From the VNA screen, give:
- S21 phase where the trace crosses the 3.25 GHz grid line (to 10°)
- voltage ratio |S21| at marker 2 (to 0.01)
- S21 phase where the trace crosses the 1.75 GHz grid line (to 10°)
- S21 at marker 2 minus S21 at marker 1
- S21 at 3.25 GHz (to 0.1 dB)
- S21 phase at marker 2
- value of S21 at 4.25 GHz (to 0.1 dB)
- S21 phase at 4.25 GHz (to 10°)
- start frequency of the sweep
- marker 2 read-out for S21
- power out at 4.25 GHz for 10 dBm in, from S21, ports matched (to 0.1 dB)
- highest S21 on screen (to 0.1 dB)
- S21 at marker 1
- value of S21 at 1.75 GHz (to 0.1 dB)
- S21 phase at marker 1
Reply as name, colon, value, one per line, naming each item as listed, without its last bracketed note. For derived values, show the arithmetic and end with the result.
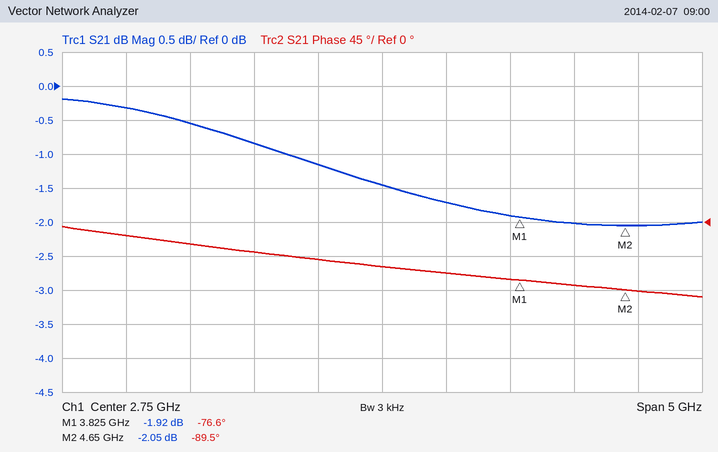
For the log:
S21 phase where the trace crosses the 3.25 GHz grid line: -70°
voltage ratio |S21| at marker 2: 10^(-2.05/20) ≈ 0.79
S21 phase where the trace crosses the 1.75 GHz grid line: -40°
S21 at marker 2 minus S21 at marker 1: -2.05 − (-1.92) = -0.13 dB
S21 at 3.25 GHz: -1.7 dB
S21 phase at marker 2: -89.5°
value of S21 at 4.25 GHz: -2.0 dB
S21 phase at 4.25 GHz: -80°
start frequency of the sweep: 250 MHz
marker 2 read-out for S21: -2.05 dB
power out at 4.25 GHz for 10 dBm in, from S21, ports matched: 10 dBm + (-2.0 dB) = 8.0 dBm
highest S21 on screen: -0.2 dB
S21 at marker 1: -1.92 dB
value of S21 at 1.75 GHz: -0.8 dB
S21 phase at marker 1: -76.6°
